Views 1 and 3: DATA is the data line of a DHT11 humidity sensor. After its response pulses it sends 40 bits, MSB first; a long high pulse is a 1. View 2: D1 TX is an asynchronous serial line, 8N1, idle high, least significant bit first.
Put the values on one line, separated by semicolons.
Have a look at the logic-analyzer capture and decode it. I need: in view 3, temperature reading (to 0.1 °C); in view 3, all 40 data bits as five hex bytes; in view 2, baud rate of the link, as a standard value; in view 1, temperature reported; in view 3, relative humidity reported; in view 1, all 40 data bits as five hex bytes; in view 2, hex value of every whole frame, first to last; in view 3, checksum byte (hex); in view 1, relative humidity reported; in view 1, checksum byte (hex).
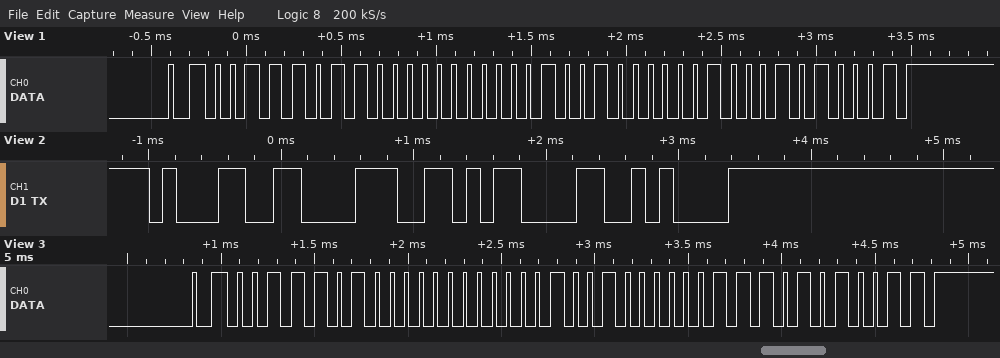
18.7 °C; 3A 00 12 07 53; 9600 baud; 18.4 °C; 58 %; 3B 00 12 04 51; 0x31 0x38 0x0D 0x0A; 0x53; 59 %; 0x51
